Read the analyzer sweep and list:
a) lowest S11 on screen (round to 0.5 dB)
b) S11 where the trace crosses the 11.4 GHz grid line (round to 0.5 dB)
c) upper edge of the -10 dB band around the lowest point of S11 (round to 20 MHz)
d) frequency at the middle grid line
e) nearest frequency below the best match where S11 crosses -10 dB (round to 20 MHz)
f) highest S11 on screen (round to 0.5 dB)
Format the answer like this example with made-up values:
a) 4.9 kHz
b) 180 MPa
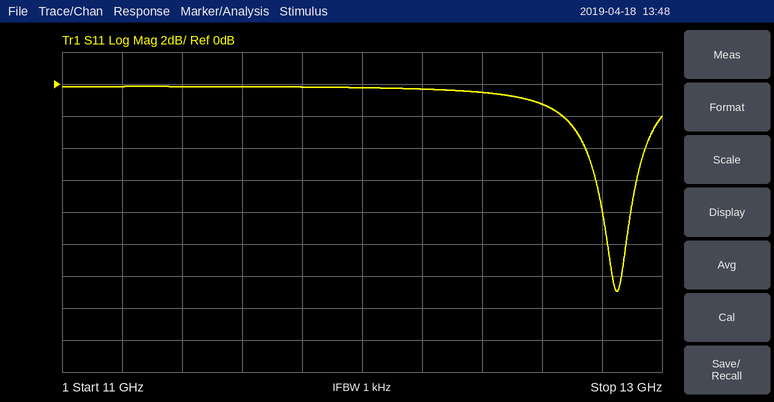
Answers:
a) -13.0 dB
b) 0.0 dB
c) 12.88 GHz
d) 12 GHz
e) 12.82 GHz
f) 0.0 dB
